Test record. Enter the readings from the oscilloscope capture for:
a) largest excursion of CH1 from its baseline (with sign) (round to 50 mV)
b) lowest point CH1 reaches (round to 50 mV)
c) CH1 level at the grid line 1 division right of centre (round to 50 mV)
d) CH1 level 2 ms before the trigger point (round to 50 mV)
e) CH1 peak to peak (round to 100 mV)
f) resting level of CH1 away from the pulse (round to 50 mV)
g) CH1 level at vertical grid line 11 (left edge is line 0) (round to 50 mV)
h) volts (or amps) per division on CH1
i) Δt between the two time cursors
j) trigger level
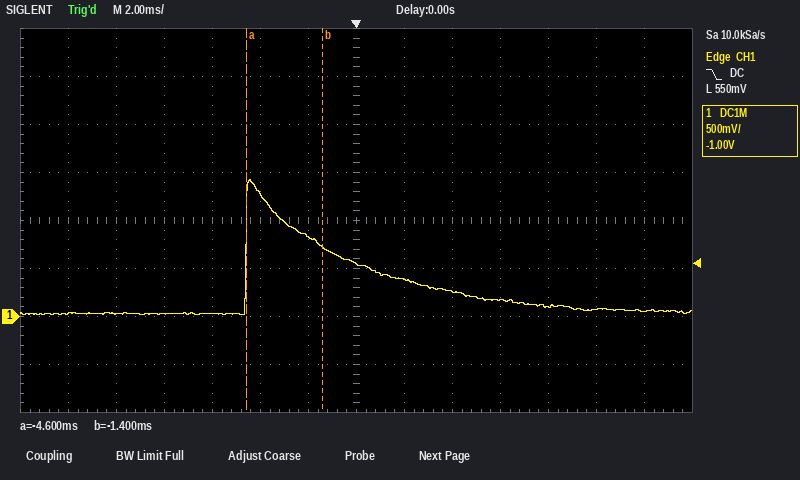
+1.40 V
0 mV
400 mV
850 mV
1.40 V
50 mV
100 mV
500 mV
3.2 ms
550 mV
